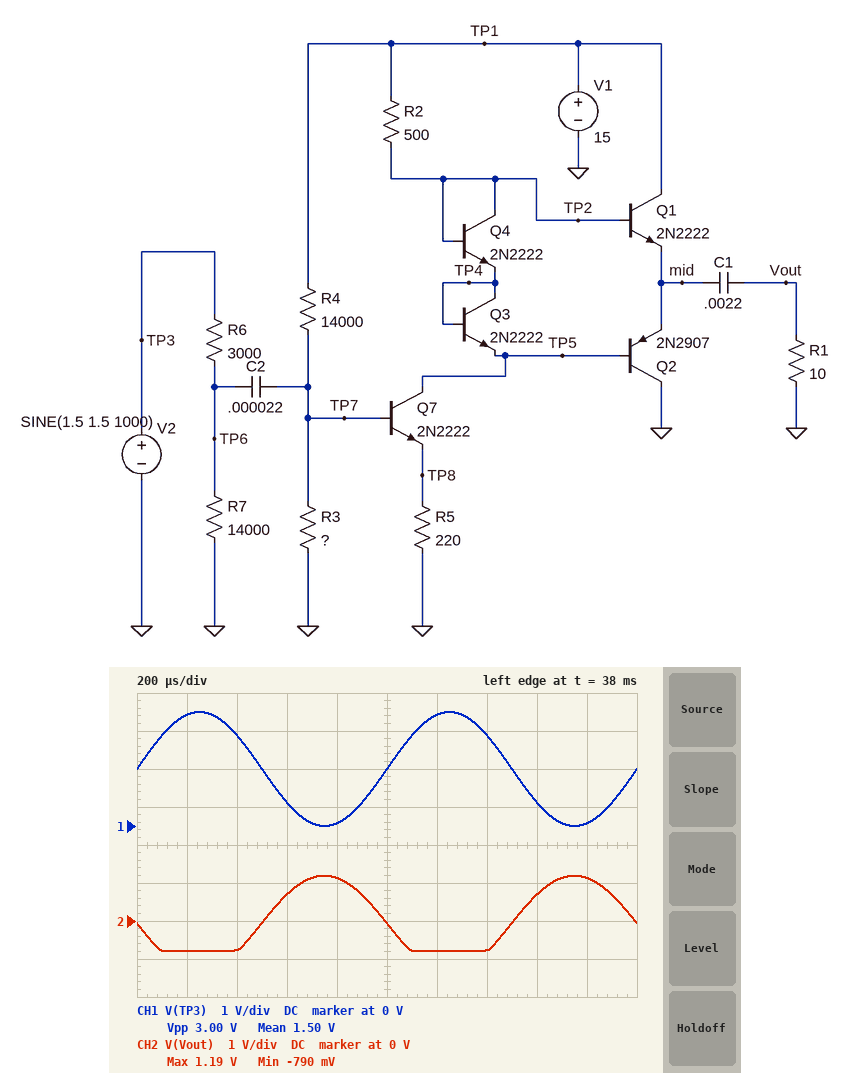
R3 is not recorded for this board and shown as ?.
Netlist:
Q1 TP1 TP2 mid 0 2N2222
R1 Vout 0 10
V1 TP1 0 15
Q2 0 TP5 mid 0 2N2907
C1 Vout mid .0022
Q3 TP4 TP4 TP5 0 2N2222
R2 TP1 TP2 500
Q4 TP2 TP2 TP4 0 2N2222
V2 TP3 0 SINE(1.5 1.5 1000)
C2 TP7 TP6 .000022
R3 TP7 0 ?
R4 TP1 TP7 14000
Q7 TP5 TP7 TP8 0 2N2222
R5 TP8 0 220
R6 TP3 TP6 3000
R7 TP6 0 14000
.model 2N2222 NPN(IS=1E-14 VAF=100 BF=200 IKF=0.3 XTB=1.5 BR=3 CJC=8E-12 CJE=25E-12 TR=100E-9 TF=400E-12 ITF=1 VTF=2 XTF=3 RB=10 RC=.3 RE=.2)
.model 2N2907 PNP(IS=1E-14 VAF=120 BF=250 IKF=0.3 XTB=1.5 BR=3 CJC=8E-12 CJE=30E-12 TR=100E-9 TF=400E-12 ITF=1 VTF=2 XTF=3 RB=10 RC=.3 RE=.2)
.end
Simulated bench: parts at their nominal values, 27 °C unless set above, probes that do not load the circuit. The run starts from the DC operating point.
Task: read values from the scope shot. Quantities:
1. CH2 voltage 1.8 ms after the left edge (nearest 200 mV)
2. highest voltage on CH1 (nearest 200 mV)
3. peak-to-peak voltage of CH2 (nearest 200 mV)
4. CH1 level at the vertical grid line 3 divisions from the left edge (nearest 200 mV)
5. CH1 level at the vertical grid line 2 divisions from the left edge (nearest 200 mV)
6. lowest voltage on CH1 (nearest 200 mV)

1.2 V
3.0 V
2.0 V
600 mV
2.4 V
0 V
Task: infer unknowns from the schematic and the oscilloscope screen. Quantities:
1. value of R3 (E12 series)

6.8 kΩ
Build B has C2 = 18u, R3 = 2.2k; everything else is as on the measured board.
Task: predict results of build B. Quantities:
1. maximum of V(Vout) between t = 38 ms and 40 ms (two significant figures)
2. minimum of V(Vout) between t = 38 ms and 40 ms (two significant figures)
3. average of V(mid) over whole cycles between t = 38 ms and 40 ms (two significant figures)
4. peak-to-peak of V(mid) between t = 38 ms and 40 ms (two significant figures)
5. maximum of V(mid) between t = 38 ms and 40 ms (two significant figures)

830 mV
-860 mV
11 V
1.7 V
12 V
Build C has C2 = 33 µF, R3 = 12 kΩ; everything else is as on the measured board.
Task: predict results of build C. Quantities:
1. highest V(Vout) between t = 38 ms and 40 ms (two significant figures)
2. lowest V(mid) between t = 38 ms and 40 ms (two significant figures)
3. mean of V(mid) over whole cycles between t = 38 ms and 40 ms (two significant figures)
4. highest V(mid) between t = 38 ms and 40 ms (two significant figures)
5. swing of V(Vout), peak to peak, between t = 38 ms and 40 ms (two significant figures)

640 mV
5.0 V
5.2 V
5.8 V
800 mV
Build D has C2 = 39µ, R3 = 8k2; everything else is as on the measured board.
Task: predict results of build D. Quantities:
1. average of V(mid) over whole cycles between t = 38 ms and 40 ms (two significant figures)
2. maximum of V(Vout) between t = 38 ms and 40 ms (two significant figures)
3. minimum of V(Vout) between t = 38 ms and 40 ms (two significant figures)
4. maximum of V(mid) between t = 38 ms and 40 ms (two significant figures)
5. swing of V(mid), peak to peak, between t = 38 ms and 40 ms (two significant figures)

5.5 V
1.0 V
-330 mV
6.4 V
1.3 V
